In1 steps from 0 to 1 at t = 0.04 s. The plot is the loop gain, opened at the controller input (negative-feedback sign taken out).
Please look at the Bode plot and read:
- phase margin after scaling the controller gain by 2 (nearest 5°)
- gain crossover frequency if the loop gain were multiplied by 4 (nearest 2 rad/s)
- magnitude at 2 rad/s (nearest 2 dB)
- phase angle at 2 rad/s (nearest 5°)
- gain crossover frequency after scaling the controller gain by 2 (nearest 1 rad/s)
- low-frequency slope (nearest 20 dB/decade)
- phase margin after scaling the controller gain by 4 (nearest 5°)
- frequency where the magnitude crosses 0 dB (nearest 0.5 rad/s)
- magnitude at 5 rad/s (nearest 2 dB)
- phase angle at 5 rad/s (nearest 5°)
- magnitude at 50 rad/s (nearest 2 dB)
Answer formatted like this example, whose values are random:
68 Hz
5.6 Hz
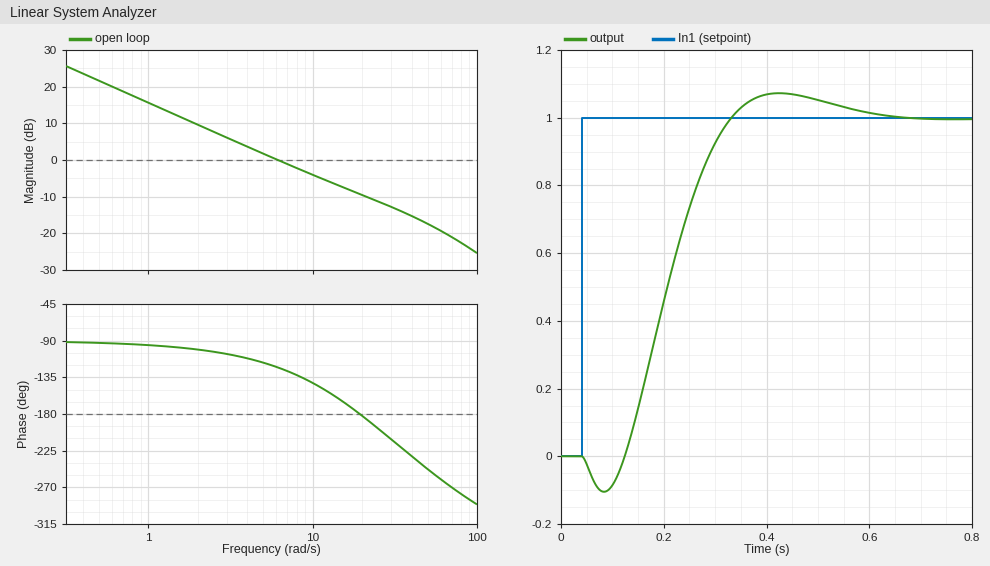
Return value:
25°
28 rad/s
10 dB
-100°
13 rad/s
-20 dB/decade
-25°
6.0 rad/s
2 dB
-115°
-18 dB
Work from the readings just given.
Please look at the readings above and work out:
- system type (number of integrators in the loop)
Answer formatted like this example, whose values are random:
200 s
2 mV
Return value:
1
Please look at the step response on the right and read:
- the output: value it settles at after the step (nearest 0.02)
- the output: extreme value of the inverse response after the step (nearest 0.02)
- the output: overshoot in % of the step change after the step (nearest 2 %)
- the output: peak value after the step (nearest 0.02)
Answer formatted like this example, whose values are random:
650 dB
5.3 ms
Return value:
1.00
-0.10
8 %
1.08
